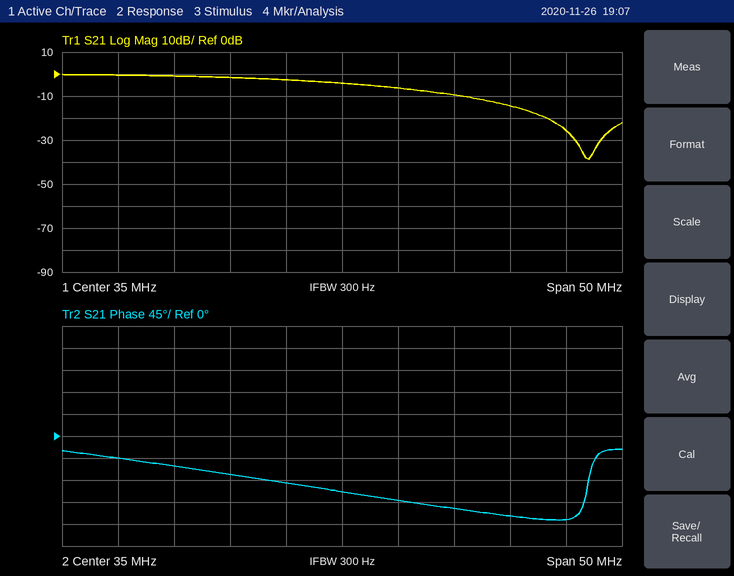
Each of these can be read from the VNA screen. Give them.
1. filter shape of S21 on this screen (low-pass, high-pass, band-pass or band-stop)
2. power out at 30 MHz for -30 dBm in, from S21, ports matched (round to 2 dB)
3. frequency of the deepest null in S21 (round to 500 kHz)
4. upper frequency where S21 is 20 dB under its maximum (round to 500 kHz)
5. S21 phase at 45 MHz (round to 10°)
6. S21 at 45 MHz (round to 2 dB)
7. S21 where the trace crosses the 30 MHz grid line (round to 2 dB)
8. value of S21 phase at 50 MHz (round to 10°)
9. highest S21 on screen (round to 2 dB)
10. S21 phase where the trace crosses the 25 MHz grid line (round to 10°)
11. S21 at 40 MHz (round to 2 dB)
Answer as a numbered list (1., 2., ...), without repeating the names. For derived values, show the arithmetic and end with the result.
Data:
1. low-pass
2. -30 dBm + (-2 dB) = -32 dBm
3. 57.0 MHz
4. 53.5 MHz
5. -150°
6. -10 dB
7. -2 dB
8. -160°
9. 0 dB
10. -80°
11. -6 dB
